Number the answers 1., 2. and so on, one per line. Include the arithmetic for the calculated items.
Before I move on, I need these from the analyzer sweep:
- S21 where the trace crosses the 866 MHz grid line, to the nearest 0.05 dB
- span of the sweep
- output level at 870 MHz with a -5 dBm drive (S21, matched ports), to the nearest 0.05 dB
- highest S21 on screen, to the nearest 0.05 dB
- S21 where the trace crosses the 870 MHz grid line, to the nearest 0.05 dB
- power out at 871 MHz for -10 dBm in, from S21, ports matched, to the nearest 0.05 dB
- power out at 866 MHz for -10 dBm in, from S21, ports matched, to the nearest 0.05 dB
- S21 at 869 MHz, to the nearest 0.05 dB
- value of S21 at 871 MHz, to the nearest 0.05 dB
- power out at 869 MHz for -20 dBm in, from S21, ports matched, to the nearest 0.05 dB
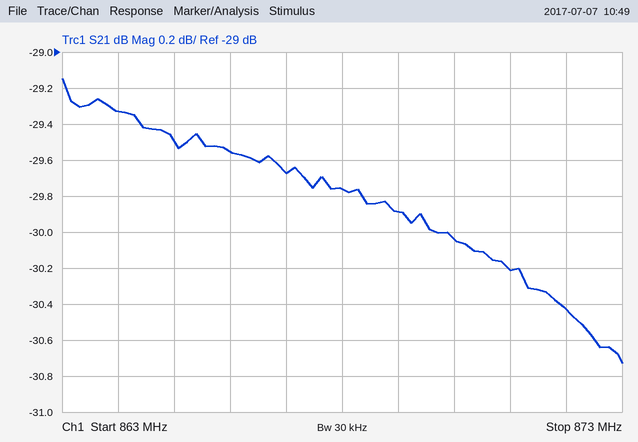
1. -29.55 dB
2. 10 MHz
3. -5 dBm + (-30.05 dB) = -35.05 dBm
4. -29.15 dB
5. -30.05 dB
6. -10 dBm + (-30.20 dB) = -40.20 dBm
7. -10 dBm + (-29.55 dB) = -39.55 dBm
8. -29.90 dB
9. -30.20 dB
10. -20 dBm + (-29.90 dB) = -49.90 dBm
